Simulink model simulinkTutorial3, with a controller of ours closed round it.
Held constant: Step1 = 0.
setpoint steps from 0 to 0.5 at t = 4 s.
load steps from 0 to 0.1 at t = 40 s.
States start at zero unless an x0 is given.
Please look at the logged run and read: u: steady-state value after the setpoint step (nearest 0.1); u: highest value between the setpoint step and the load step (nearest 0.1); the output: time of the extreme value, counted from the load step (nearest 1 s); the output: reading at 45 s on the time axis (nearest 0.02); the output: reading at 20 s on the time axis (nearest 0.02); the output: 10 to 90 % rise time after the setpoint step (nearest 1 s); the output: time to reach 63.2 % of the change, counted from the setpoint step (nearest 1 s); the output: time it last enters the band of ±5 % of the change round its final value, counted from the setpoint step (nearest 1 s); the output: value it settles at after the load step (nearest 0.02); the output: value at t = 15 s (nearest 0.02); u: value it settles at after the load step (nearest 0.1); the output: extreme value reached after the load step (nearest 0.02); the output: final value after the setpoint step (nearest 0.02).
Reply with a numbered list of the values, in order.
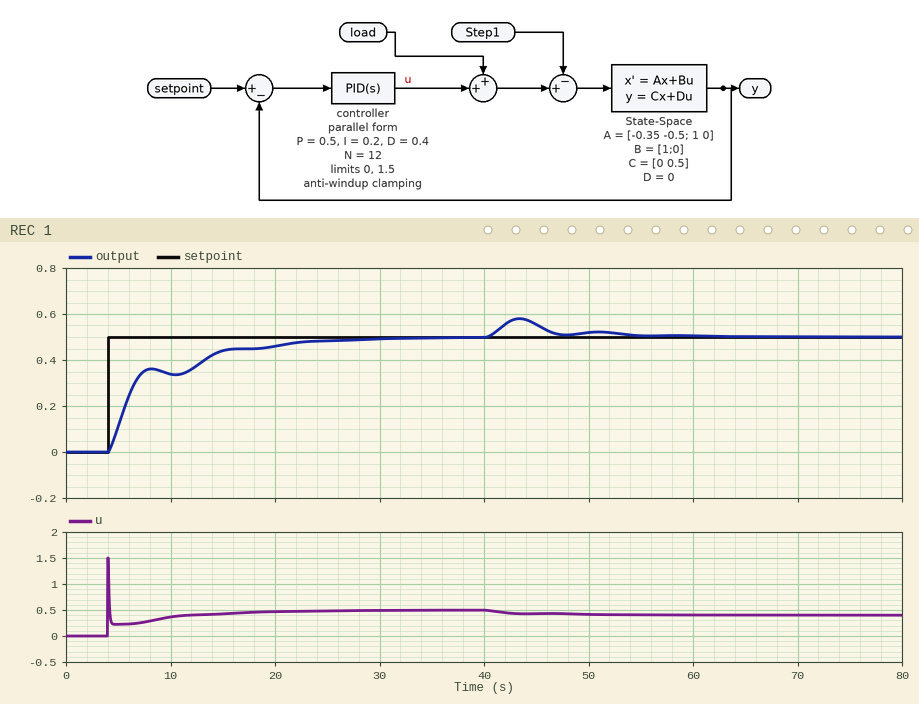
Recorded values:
1. 0.5
2. 1.5
3. 3 s
4. 0.56
5. 0.46
6. 14 s
7. 3 s
8. 18 s
9. 0.50
10. 0.44
11. 0.4
12. 0.58
13. 0.50
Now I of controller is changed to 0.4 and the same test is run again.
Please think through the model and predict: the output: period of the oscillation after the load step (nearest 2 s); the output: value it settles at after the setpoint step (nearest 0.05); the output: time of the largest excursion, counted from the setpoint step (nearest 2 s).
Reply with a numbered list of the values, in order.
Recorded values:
1. 8 s
2. 0.50
3. 12 s
